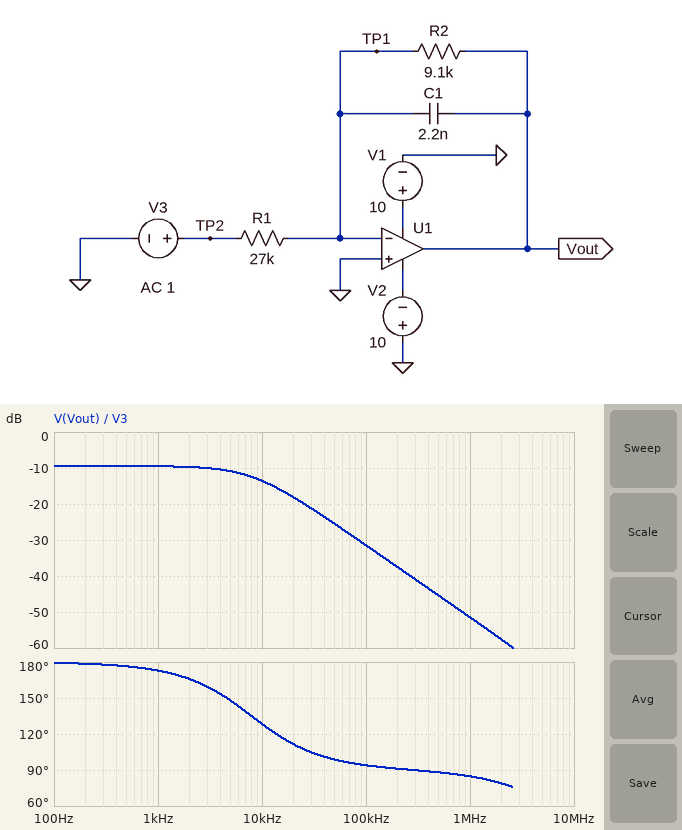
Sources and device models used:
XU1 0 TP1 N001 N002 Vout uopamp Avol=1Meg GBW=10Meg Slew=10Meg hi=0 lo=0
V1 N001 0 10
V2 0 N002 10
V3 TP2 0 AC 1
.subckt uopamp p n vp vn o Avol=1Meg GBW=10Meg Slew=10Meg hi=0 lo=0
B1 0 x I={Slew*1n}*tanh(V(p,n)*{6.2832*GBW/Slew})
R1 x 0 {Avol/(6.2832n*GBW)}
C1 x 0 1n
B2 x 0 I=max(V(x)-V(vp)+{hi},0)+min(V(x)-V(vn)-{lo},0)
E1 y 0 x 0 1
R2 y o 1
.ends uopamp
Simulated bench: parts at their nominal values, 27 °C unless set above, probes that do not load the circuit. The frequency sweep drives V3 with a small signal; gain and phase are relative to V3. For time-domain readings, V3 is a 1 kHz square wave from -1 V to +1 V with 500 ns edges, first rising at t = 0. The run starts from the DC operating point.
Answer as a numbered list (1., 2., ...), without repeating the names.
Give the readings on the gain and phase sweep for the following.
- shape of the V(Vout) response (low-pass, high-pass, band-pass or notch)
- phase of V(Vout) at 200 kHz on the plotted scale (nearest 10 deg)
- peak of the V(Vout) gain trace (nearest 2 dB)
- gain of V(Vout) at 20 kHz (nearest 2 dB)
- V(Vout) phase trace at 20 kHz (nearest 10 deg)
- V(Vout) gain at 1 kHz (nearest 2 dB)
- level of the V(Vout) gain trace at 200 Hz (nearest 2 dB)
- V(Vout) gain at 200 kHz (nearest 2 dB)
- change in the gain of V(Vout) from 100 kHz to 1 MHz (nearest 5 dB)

1. low-pass
2. 90 deg
3. -10 dB
4. -18 dB
5. 110 deg
6. -10 dB
7. -10 dB
8. -38 dB
9. -20 dB
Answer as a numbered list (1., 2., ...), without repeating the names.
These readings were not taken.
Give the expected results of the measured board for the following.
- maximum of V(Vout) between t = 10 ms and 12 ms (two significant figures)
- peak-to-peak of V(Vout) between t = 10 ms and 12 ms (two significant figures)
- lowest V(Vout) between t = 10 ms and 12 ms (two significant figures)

1. 340 mV
2. 670 mV
3. -340 mV
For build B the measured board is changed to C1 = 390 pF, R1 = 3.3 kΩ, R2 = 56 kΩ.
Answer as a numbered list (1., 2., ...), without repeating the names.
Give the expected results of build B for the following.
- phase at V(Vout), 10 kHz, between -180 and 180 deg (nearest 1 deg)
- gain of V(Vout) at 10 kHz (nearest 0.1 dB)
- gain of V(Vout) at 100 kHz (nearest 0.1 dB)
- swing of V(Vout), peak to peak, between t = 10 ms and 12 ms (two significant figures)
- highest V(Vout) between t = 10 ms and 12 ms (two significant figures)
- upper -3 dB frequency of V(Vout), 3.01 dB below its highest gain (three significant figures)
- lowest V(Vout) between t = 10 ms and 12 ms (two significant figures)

1. 126 deg
2. 19.9 dB
3. 1.7 dB
4. 20 V
5. 10 V
6. 7.20 kHz
7. -10 V
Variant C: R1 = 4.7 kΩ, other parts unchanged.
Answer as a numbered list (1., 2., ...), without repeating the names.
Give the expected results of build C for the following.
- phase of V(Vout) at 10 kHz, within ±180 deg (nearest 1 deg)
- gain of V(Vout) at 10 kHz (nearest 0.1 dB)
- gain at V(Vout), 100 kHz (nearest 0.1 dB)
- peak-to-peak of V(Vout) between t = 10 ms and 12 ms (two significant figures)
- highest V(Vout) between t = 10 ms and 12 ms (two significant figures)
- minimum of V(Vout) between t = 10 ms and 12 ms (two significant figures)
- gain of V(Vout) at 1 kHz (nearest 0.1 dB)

1. 128 deg
2. 1.6 dB
3. -16.3 dB
4. 3.9 V
5. 1.9 V
6. -1.9 V
7. 5.7 dB
